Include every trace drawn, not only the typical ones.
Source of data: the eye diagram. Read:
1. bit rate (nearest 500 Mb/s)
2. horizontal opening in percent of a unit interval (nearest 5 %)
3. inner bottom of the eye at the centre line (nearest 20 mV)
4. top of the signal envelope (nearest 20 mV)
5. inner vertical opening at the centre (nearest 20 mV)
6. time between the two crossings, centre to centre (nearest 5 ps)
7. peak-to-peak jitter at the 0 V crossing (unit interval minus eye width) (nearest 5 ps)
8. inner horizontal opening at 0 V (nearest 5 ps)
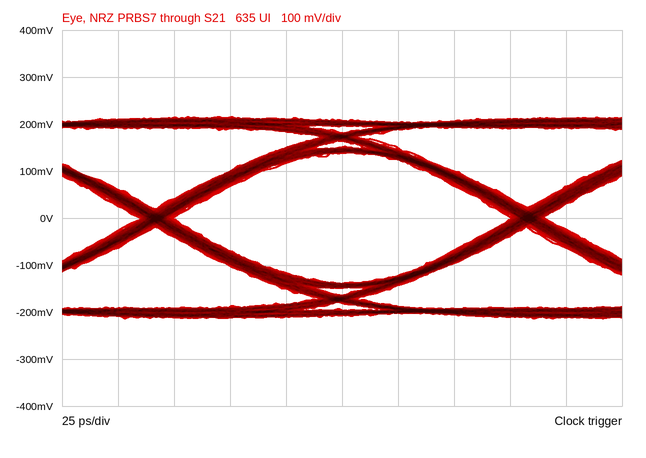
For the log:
6.0 Gb/s
90 %
-140 mV
220 mV
280 mV
165 ps
15 ps
150 ps
